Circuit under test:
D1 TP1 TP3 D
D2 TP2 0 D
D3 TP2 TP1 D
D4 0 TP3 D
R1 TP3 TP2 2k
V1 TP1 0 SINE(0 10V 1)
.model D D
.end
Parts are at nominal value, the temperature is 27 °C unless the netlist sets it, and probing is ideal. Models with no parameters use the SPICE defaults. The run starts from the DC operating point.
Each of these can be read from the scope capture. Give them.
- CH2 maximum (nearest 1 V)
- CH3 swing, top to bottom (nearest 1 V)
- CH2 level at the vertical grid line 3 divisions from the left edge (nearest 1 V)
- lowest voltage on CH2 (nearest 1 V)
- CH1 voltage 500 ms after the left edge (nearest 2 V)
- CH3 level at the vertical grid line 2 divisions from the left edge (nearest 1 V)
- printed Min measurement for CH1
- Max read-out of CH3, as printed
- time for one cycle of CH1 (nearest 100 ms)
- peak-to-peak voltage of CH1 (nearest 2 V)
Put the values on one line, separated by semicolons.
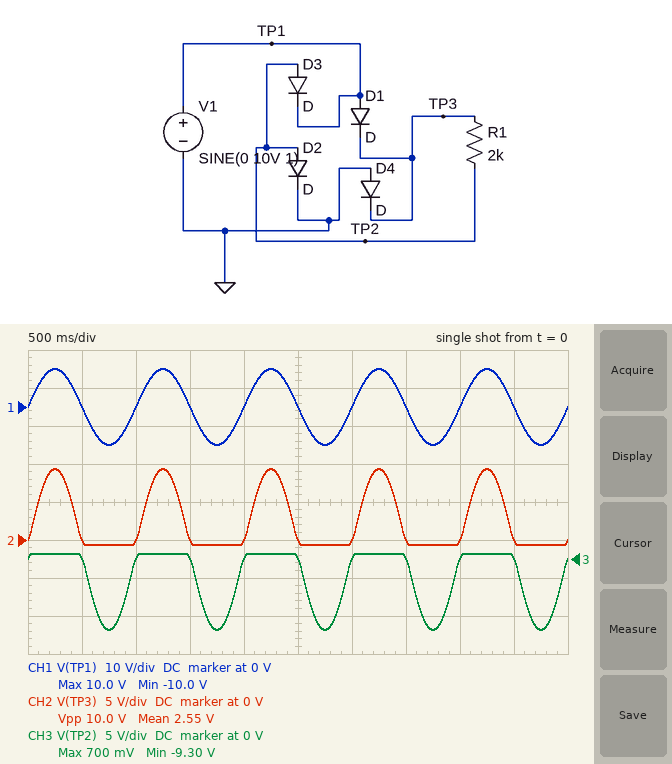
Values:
9 V; 10 V; 0 V; -1 V; 0 V; 0 V; -10.0 V; 700 mV; 1.0 s; 20 V
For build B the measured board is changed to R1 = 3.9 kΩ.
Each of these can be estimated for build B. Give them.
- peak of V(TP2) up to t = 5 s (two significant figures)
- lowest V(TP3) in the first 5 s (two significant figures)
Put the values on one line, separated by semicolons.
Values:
680 mV; -680 mV
